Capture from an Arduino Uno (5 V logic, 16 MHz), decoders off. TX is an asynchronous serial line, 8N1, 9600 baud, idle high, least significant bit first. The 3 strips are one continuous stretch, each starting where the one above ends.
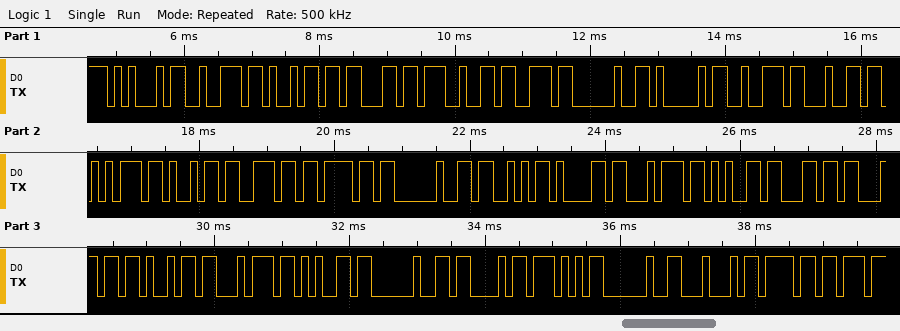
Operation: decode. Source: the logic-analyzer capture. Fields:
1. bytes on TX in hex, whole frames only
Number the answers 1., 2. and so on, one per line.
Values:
1. 45 72 69 63 27 73 20 41 72 64 75 69 6E 6F 20 53 61 74 65 6C 6C 69 74 65 20 43 57 20 44 6F
